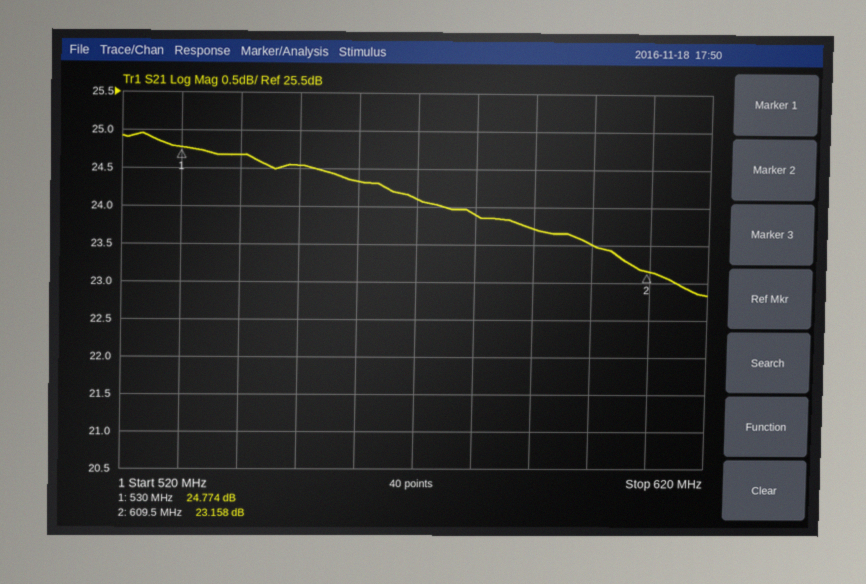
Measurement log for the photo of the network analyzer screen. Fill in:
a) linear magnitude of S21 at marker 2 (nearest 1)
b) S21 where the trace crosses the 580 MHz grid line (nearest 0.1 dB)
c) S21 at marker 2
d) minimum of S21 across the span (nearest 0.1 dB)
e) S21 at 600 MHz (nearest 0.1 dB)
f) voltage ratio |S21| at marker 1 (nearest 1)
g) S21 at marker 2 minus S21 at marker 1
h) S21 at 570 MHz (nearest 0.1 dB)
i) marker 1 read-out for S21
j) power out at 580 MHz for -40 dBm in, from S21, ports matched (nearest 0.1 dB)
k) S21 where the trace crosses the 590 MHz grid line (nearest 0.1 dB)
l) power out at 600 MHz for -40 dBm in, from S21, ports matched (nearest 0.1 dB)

14
23.9 dB
23.158 dB
22.8 dB
23.5 dB
17
-1.616 dB
24.1 dB
24.774 dB
-16.1 dBm
23.7 dB
-16.5 dBm
